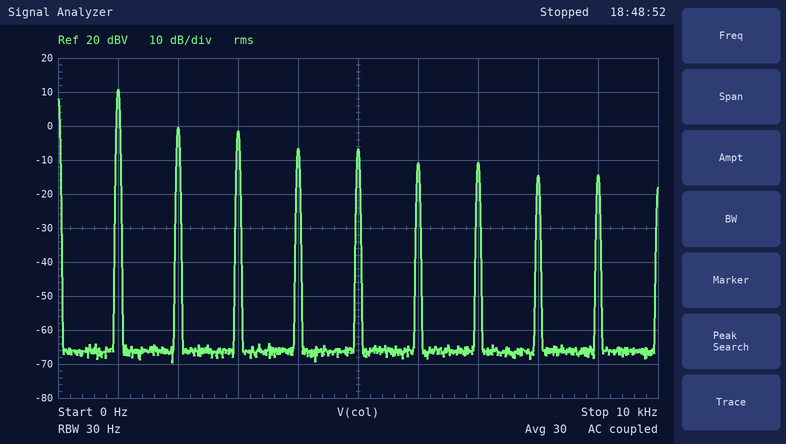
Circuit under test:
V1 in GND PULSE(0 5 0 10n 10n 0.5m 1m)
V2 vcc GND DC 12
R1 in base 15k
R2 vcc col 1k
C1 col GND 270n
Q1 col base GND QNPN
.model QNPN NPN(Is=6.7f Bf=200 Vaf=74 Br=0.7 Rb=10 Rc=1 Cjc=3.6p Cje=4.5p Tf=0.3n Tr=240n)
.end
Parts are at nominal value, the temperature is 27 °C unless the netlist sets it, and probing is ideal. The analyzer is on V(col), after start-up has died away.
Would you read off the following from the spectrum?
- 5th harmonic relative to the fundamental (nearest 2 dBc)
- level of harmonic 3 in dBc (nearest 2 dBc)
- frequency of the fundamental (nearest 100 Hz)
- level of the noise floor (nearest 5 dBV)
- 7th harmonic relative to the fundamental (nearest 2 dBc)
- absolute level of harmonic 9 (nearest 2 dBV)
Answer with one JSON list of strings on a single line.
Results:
["-18 dBc", "-12 dBc", "1.0 kHz", "-65 dBV", "-22 dBc", "-14 dBV"]
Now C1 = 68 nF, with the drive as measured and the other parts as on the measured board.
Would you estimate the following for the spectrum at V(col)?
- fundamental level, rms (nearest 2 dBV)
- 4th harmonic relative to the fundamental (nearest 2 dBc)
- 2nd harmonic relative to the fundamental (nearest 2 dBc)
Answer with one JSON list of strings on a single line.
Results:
["14 dBV", "-20 dBc", "-16 dBc"]
